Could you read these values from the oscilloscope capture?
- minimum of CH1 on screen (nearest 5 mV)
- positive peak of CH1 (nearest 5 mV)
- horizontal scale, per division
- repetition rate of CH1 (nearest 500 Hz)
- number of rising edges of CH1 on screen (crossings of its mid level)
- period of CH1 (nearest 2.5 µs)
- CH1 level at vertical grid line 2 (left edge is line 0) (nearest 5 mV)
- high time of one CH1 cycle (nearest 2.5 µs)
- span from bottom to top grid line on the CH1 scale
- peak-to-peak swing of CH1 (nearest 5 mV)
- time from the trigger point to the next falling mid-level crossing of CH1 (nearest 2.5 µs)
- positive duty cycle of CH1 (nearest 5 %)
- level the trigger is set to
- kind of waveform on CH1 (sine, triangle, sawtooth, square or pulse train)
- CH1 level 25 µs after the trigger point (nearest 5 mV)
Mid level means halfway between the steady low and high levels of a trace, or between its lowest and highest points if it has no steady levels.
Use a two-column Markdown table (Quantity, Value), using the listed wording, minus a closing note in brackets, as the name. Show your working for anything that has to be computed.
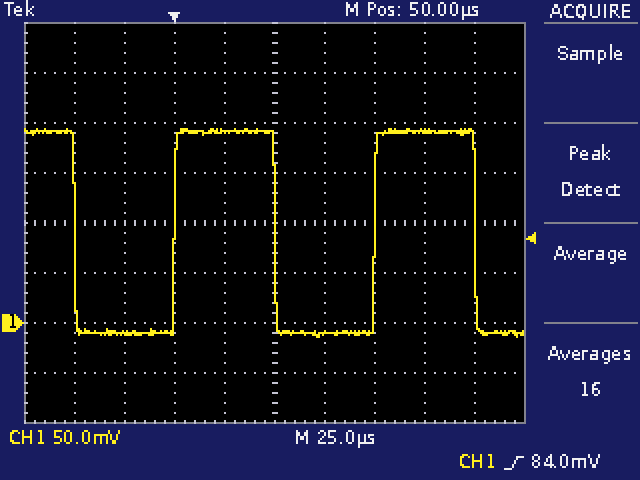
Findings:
| Quantity | Value |
|---|---|
| minimum of CH1 on screen | -15 mV |
| positive peak of CH1 | 195 mV |
| horizontal scale, per division | 25 µs |
| repetition rate of CH1 | 1 / 100.0 µs ≈ 10.0 kHz |
| number of rising edges of CH1 on screen | 2 |
| period of CH1 | 100.0 µs |
| CH1 level at vertical grid line 2 (left edge is line 0) | -10 mV |
| high time of one CH1 cycle | 50.0 µs |
| span from bottom to top grid line on the CH1 scale | 400 mV |
| peak-to-peak swing of CH1 | 195 mV − (-15 mV) = 210 mV |
| time from the trigger point to the next falling mid-level crossing of CH1 | 50.0 µs |
| positive duty cycle of CH1 | 50.0 µs / 100.0 µs ≈ 50 % |
| level the trigger is set to | 84.0 mV |
| kind of waveform on CH1 | square |
| CH1 level 25 µs after the trigger point | 190 mV |
